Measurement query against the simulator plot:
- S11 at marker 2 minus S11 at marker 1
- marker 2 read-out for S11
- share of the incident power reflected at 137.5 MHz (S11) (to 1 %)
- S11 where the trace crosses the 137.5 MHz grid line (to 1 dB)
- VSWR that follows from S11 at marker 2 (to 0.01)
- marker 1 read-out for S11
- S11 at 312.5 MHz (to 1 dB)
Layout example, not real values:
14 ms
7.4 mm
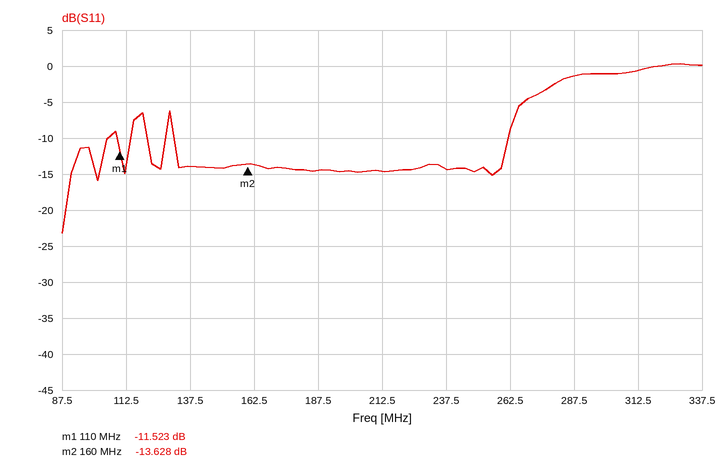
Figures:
-2.105 dB
-13.628 dB
4 %
-14 dB
1.53
-11.523 dB
-1 dB
